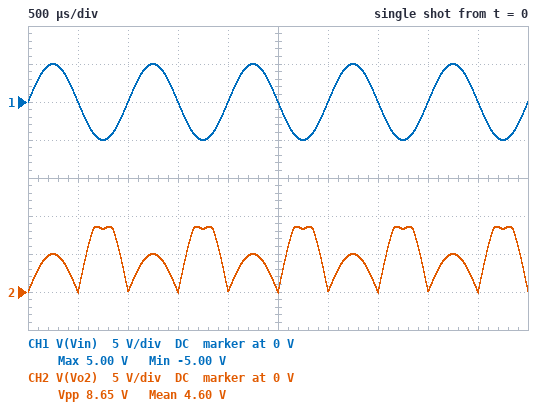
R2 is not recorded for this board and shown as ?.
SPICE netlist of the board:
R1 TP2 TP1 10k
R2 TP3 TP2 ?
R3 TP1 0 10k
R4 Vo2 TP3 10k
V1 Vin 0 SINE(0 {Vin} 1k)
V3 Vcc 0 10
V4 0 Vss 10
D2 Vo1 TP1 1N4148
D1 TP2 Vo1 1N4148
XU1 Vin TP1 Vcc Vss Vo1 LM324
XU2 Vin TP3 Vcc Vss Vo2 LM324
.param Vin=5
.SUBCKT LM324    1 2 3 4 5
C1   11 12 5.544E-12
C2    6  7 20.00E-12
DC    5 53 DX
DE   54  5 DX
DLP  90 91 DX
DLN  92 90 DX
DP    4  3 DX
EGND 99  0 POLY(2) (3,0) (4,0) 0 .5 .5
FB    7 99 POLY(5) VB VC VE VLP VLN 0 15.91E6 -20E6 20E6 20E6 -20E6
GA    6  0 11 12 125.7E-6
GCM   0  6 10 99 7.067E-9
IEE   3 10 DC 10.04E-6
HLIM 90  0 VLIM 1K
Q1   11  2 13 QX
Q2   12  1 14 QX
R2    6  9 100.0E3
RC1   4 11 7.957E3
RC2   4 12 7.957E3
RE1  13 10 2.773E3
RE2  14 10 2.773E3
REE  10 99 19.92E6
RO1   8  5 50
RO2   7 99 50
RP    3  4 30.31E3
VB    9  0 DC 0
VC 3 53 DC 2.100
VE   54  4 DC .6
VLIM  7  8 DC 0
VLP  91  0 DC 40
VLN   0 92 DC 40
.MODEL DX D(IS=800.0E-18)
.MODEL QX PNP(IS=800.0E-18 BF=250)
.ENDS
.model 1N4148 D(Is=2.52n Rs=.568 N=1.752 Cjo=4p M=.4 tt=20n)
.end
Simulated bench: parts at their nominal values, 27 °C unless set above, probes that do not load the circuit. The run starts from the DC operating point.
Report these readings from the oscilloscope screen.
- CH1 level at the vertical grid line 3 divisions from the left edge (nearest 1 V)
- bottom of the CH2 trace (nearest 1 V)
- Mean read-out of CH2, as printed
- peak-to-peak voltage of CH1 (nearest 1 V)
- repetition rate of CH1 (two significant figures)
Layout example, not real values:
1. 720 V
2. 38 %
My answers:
1. 0 V
2. 0 V
3. 4.60 V
4. 10 V
5. 1.0 kHz
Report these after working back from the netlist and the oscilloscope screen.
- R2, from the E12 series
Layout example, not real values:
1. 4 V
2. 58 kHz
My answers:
1. 3.3 kΩ
